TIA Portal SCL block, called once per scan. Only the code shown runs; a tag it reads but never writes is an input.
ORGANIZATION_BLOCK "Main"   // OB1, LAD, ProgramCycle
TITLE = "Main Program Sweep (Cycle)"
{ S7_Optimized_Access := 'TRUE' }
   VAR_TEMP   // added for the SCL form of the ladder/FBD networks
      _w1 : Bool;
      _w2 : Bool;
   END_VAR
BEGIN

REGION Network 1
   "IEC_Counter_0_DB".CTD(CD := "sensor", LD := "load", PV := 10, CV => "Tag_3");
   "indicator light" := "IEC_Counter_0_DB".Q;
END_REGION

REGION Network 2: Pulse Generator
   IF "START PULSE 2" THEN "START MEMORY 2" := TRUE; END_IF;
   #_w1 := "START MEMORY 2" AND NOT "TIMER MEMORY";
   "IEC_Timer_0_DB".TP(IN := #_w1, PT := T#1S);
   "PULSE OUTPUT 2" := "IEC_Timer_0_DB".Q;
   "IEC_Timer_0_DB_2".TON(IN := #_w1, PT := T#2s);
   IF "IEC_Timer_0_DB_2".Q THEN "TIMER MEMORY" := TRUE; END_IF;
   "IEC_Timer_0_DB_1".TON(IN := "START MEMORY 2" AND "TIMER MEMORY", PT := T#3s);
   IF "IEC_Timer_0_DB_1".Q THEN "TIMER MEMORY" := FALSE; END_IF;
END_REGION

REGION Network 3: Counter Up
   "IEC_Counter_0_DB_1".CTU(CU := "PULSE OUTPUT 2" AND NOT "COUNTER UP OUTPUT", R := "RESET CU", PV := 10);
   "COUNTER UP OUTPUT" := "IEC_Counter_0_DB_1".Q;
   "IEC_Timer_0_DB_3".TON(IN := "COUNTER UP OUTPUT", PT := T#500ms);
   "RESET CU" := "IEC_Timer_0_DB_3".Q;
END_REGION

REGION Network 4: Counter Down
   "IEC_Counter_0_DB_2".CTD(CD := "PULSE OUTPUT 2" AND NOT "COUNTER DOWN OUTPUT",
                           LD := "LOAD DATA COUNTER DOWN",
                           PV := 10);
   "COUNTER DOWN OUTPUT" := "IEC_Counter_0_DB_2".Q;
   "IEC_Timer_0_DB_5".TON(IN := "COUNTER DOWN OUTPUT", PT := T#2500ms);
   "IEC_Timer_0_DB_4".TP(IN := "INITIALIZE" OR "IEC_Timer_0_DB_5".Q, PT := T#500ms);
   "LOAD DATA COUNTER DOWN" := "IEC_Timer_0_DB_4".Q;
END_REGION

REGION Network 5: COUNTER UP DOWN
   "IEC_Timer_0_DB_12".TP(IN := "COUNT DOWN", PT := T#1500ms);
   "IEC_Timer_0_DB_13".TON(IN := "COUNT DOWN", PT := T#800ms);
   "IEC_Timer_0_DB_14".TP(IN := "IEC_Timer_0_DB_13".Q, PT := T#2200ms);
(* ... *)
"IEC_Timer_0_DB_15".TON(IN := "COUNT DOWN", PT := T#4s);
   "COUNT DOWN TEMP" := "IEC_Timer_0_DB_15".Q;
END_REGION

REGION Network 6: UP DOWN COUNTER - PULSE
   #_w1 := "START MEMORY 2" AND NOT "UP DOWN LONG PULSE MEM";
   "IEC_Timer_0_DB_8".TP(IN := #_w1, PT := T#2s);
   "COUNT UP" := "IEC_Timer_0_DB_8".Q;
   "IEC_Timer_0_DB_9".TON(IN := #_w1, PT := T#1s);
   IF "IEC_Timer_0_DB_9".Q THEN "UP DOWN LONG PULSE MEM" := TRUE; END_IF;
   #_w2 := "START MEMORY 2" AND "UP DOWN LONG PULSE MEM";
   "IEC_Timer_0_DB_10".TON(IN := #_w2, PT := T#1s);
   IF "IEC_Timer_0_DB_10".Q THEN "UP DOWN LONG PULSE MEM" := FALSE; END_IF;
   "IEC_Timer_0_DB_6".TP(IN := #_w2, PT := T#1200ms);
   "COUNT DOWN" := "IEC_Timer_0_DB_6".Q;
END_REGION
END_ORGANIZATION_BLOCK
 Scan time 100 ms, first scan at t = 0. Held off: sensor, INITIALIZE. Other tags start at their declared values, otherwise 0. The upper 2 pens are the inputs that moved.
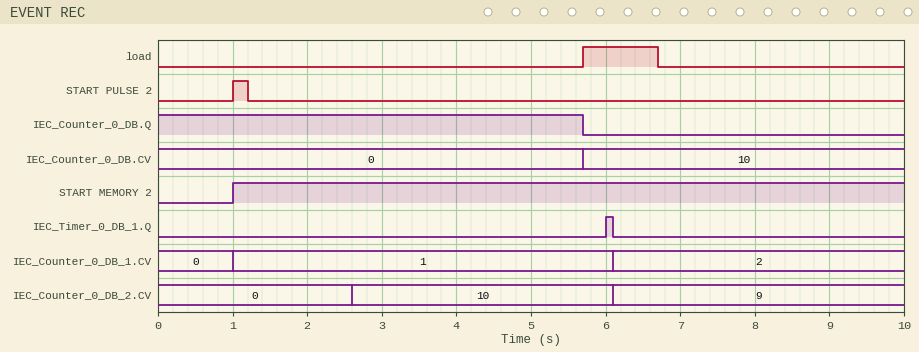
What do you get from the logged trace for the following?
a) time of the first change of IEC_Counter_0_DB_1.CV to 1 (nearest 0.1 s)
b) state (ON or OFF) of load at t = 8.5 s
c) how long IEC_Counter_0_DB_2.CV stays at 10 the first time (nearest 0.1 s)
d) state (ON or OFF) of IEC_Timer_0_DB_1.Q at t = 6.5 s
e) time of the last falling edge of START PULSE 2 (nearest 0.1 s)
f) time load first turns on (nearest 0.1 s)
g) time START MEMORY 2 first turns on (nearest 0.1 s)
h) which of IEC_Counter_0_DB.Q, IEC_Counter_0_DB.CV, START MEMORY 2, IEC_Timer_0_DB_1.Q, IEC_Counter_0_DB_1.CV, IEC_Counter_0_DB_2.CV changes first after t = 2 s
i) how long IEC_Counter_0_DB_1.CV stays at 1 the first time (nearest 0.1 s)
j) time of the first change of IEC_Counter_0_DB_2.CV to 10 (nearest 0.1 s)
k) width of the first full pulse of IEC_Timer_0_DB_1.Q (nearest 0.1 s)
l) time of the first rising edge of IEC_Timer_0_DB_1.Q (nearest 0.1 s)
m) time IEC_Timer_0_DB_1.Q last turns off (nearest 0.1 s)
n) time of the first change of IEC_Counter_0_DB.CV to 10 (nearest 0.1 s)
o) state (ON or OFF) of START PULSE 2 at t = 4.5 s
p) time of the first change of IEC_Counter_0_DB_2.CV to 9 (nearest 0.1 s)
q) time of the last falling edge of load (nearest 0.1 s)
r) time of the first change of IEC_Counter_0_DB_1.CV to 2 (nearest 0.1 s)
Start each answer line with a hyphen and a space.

- 1.0 s
- OFF
- 3.5 s
- OFF
- 1.2 s
- 5.7 s
- 1.0 s
- IEC_Counter_0_DB_2.CV
- 5.1 s
- 2.6 s
- 0.1 s
- 6.0 s
- 6.1 s
- 5.7 s
- OFF
- 6.1 s
- 6.7 s
- 6.1 s
